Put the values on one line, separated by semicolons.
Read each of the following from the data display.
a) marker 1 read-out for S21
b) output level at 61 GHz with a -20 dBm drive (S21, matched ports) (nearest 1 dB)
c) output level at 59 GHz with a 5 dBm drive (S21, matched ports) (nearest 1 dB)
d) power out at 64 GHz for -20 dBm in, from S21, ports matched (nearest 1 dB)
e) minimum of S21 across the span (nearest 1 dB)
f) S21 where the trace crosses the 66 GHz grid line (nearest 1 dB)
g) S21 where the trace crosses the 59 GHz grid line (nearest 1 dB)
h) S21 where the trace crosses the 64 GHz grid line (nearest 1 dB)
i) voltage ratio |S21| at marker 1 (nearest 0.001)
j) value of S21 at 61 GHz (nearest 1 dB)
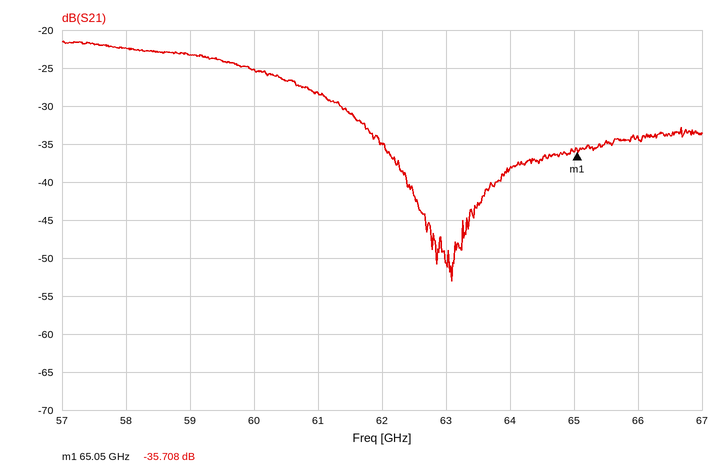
-35.708 dB; -48 dBm; -18 dBm; -58 dBm; -53 dB; -34 dB; -23 dB; -38 dB; 0.016; -28 dB
